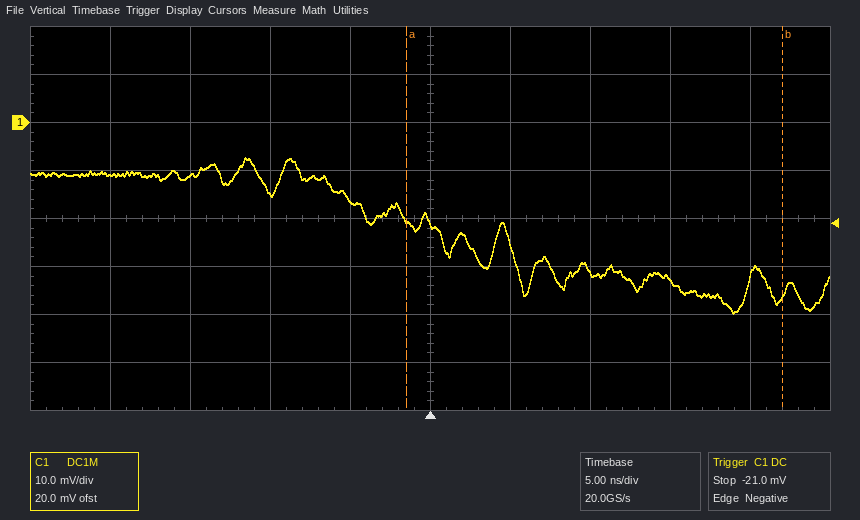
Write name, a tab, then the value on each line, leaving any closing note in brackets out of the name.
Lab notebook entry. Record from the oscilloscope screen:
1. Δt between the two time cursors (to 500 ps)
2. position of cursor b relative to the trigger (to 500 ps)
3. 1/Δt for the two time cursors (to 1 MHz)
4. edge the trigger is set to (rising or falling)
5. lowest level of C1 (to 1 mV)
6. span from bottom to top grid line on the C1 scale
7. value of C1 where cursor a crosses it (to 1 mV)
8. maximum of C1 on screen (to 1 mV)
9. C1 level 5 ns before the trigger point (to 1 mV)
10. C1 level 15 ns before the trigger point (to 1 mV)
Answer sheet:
Δt between the two time cursors	23.5 ns
position of cursor b relative to the trigger	+22.0 ns
1/Δt for the two time cursors	43 MHz
edge the trigger is set to	falling
lowest level of C1	-40 mV
span from bottom to top grid line on the C1 scale	80 mV
value of C1 where cursor a crosses it	-20 mV
maximum of C1 on screen	-7 mV
C1 level 5 ns before the trigger point	-16 mV
C1 level 15 ns before the trigger point	-11 mV
